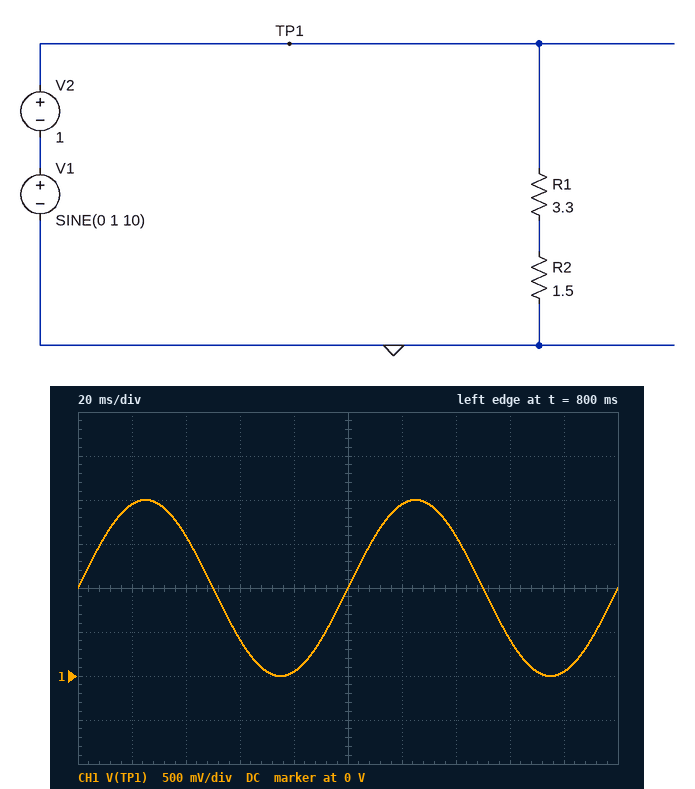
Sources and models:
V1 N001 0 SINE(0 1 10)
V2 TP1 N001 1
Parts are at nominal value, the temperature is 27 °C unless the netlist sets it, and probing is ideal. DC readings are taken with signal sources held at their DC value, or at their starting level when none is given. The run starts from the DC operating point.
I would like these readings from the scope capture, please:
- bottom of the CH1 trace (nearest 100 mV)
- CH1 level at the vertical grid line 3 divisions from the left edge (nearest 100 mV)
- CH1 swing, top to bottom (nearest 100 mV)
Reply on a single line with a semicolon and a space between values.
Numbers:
0 V; 400 mV; 2.0 V
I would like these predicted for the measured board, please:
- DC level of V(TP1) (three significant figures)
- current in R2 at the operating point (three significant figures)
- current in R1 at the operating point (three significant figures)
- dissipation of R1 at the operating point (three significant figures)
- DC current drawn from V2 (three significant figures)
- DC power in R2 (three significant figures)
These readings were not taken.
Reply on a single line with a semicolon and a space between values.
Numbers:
1.00 V; 208 mA; 208 mA; 143 mW; 208 mA; 65.1 mW
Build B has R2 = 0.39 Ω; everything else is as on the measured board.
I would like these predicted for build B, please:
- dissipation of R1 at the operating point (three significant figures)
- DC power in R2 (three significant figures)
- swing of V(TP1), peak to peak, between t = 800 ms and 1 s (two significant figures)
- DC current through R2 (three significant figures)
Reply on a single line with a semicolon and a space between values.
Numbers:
242 mW; 28.6 mW; 2.0 V; 271 mA
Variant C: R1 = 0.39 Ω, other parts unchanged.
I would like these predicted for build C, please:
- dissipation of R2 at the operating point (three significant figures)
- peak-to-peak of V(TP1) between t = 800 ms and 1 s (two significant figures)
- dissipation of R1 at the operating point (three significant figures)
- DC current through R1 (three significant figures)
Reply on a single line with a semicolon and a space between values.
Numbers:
420 mW; 2.0 V; 109 mW; 529 mA
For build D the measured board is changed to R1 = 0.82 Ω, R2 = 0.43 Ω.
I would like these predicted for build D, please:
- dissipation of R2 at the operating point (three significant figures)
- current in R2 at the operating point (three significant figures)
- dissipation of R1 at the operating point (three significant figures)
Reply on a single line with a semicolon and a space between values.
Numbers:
275 mW; 800 mA; 525 mW
